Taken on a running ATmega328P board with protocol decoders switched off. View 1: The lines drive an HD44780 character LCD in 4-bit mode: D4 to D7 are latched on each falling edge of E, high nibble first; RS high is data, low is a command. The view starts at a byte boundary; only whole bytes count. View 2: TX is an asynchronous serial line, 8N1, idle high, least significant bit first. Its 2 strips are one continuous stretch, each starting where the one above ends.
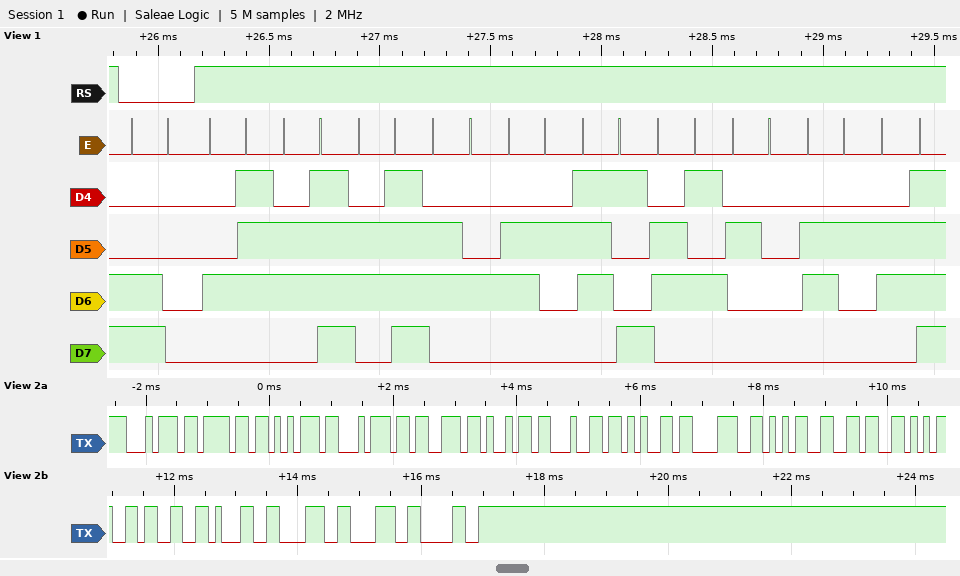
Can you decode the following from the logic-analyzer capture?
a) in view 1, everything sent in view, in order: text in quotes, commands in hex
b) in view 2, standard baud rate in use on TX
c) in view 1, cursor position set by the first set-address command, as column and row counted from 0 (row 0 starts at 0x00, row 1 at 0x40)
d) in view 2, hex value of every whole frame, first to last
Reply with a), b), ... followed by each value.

a) 0xC0 "Goodbye bo"
b) 9600 baud
c) column 0, row 1
d) 74 6F 75 74 73 69 64 65 38 35 36 35 33 31 38 38 30
